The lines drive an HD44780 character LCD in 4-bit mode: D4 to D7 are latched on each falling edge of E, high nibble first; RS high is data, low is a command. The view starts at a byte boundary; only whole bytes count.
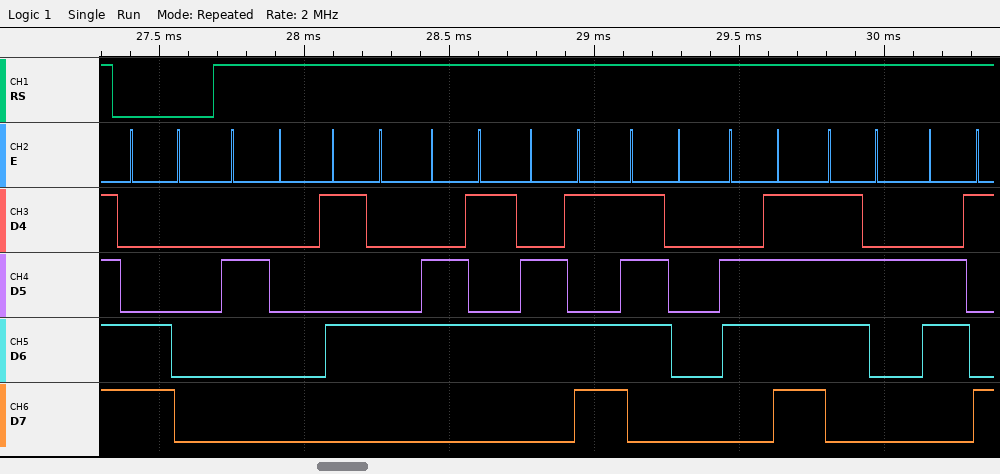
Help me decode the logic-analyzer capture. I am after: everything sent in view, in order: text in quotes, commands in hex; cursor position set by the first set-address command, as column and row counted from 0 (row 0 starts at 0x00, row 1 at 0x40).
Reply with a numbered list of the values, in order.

1. 0xC0 " Tempori"
2. column 0, row 1
